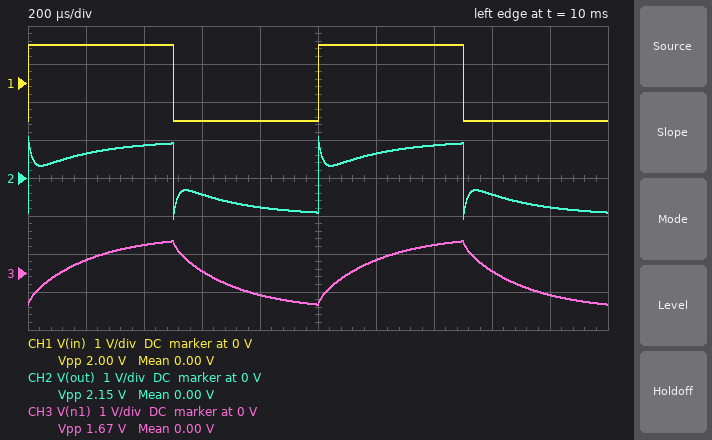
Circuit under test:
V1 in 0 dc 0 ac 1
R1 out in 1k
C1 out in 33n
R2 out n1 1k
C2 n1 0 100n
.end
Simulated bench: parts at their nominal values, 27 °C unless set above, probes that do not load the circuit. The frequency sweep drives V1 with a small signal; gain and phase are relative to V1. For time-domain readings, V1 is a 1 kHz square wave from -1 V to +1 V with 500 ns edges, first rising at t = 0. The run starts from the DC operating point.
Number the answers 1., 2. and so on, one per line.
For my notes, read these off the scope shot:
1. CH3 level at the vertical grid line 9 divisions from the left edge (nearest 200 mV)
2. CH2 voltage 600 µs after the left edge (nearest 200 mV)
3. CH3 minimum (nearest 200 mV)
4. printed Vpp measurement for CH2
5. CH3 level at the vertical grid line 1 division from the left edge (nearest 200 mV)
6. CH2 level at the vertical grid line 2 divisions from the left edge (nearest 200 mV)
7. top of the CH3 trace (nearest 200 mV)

1. -600 mV
2. -400 mV
3. -800 mV
4. 2.15 V
5. 400 mV
6. 800 mV
7. 800 mV
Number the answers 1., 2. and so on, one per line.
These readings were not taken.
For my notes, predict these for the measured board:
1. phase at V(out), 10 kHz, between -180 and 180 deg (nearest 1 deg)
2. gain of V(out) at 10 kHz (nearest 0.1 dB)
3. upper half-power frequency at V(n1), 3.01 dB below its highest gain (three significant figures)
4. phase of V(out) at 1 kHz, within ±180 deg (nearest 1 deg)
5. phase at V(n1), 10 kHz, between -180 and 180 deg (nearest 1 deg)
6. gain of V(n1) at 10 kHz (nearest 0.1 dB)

1. 16 deg
2. -2.2 dB
3. 744 Hz
4. -15 deg
5. -65 deg
6. -18.3 dB
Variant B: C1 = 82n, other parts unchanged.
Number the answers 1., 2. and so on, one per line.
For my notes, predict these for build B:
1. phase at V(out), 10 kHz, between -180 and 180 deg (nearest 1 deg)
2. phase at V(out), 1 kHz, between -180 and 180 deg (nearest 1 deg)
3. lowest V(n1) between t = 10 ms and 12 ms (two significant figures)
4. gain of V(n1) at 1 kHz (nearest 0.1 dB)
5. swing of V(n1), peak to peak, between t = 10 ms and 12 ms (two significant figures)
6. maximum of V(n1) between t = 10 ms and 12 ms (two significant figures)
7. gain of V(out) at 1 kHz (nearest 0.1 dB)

1. 9 deg
2. -10 deg
3. -820 mV
4. -4.5 dB
5. 1.6 V
6. 820 mV
7. -3.1 dB
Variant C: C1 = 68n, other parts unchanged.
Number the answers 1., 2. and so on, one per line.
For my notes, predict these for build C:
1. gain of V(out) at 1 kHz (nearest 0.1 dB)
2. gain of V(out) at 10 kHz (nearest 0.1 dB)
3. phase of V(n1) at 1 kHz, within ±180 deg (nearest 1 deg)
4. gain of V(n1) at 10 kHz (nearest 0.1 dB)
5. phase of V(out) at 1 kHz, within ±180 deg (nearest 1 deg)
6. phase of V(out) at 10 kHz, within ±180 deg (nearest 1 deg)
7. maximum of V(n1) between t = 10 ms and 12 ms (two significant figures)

1. -3.1 dB
2. -0.9 dB
3. -43 deg
4. -16.9 dB
5. -11 deg
6. 11 deg
7. 820 mV
